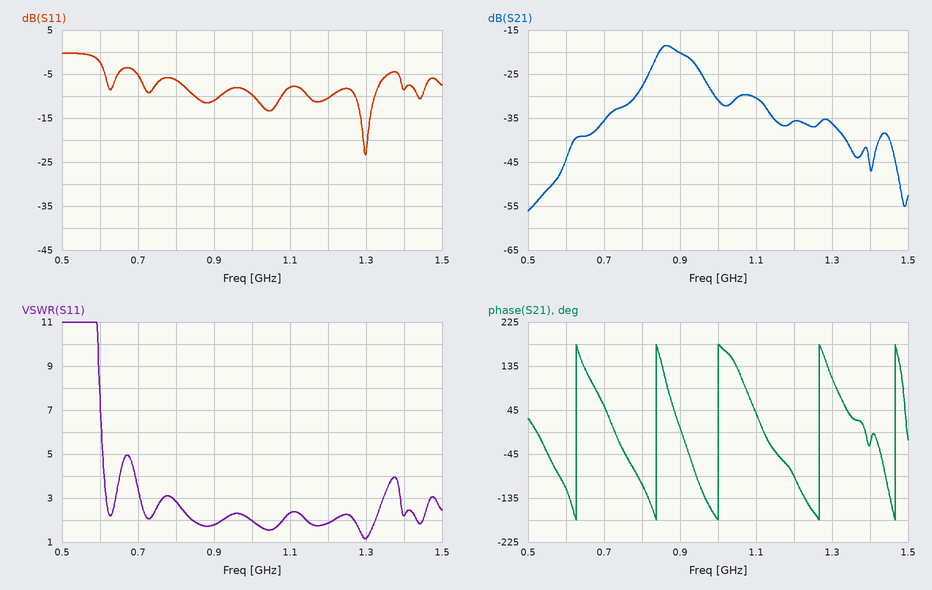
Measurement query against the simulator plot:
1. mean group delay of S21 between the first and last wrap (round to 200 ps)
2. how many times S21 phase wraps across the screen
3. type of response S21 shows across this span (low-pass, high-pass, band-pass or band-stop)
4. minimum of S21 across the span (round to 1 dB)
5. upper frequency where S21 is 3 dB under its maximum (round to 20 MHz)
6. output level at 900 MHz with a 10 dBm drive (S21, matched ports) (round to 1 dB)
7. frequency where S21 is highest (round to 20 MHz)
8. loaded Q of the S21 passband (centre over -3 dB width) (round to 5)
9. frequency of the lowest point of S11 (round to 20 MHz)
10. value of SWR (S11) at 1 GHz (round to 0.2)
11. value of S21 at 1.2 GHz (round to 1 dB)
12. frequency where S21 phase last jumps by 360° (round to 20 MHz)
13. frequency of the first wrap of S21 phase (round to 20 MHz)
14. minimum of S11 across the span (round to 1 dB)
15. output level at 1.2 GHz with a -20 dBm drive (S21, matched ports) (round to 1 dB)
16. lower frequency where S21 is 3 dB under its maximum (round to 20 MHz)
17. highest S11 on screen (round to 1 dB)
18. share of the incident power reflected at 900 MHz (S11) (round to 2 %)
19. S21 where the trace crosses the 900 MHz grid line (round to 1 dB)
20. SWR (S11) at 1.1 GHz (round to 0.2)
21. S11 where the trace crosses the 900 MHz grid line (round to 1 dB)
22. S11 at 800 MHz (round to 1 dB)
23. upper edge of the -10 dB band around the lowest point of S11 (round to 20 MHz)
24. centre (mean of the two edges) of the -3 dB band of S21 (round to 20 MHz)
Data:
4.8 ns
5
band-pass
-56 dB
920 MHz
-10 dBm
860 MHz
10
1.30 GHz
2.0
-36 dB
1.46 GHz
620 MHz
-23 dB
-56 dBm
840 MHz
0 dB
8 %
-20 dB
2.4
-11 dB
-6 dB
1.32 GHz
880 MHz
